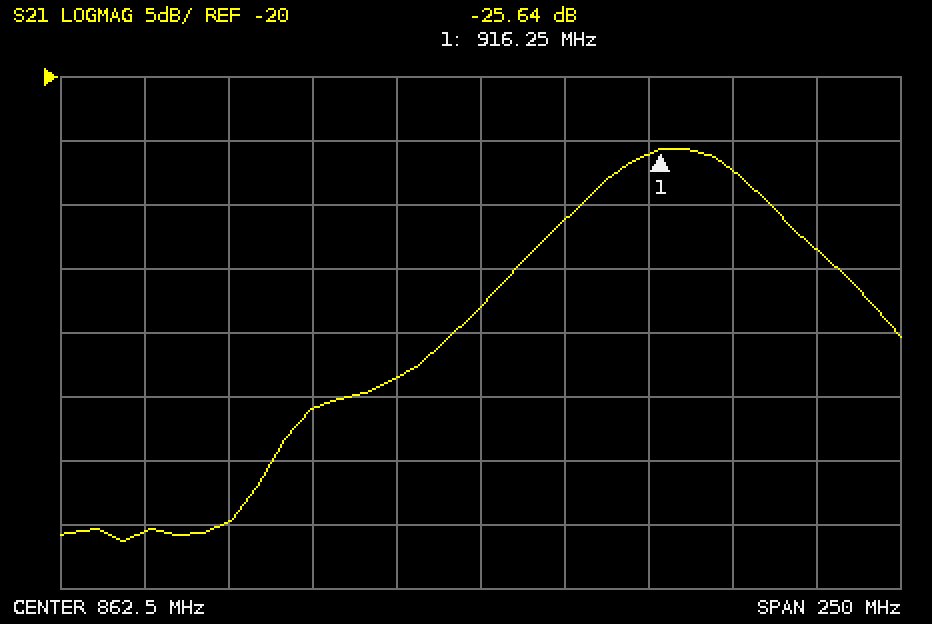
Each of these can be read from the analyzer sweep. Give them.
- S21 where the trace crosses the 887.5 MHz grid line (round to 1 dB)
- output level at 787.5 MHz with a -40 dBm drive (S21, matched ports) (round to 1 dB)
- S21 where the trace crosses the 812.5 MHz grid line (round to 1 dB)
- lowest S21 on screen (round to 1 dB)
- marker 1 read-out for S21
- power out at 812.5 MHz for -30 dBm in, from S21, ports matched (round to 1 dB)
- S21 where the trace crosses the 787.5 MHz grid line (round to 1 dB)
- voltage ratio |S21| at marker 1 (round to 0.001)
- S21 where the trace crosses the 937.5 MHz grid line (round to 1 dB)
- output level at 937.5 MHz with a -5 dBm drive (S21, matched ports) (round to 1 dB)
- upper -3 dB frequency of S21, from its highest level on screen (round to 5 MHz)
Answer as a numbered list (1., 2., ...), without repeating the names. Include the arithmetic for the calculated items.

1. -31 dB
2. -40 dBm + (-55 dB) = -95 dBm
3. -46 dB
4. -56 dB
5. -25.64 dB
6. -30 dBm + (-46 dB) = -76 dBm
7. -55 dB
8. 10^(-25.64/20) ≈ 0.052
9. -27 dB
10. -5 dBm + (-27 dB) = -32 dBm
11. 945 MHz
